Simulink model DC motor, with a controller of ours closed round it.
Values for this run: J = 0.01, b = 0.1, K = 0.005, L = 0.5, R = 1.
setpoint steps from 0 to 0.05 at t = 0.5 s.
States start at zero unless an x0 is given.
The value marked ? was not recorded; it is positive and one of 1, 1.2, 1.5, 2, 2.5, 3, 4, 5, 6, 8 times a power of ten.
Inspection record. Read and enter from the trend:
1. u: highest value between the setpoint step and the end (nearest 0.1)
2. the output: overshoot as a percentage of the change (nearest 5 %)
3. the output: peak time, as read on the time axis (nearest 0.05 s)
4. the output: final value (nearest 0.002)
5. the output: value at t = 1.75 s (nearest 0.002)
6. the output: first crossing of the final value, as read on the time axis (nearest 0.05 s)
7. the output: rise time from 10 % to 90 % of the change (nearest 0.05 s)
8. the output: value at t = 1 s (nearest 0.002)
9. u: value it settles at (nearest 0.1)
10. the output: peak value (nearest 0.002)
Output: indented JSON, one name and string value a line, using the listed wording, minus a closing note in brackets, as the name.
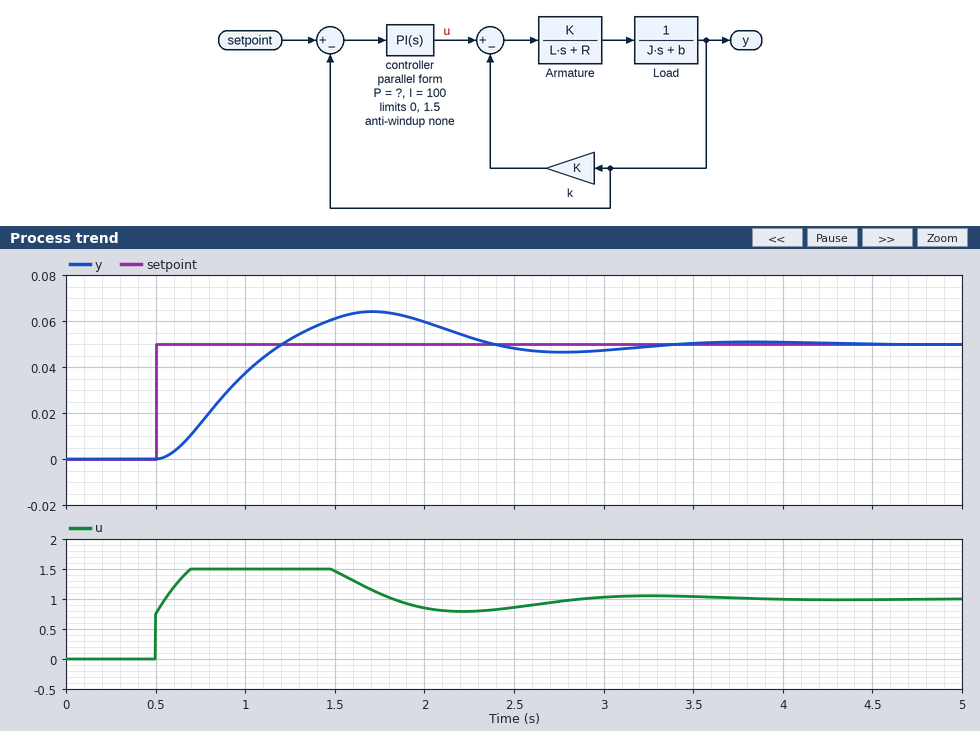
{
  "u: highest value between the setpoint step and the end": "1.5",
  "the output: overshoot as a percentage of the change": "30 %",
  "the output: peak time, as read on the time axis": "1.70 s",
  "the output: final value": "0.050",
  "the output: value at t = 1.75 s": "0.064",
  "the output: first crossing of the final value, as read on the time axis": "1.20 s",
  "the output: rise time from 10 % to 90 % of the change": "0.50 s",
  "the output: value at t = 1 s": "0.038",
  "u: value it settles at": "1.0",
  "the output: peak value": "0.064"
}
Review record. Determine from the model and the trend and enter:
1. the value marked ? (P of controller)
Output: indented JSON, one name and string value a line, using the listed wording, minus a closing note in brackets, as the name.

{
  "the value marked ?": "15"
}
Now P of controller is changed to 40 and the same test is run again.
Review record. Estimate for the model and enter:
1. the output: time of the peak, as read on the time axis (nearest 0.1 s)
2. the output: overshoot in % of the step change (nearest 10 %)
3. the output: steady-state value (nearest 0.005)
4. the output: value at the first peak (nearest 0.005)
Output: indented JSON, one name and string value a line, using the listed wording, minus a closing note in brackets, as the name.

{
  "the output: time of the peak, as read on the time axis": "1.5 s",
  "the output: overshoot in % of the step change": "20 %",
  "the output: steady-state value": "0.050",
  "the output: value at the first peak": "0.060"
}
